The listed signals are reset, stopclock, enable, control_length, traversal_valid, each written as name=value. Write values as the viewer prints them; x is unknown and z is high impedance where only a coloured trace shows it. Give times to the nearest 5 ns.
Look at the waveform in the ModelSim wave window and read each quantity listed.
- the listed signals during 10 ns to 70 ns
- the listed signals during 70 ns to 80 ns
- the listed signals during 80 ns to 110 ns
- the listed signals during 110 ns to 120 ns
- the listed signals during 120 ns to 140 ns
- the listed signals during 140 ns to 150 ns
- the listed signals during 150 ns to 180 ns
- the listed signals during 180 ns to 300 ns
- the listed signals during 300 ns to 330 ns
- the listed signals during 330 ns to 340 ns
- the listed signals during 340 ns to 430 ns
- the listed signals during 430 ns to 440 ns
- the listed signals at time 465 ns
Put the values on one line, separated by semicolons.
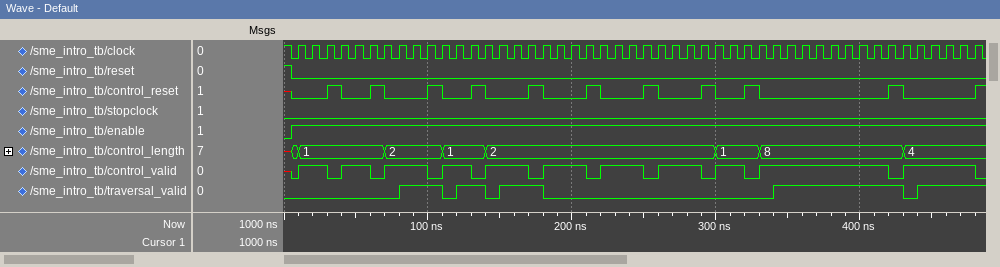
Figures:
reset=0, stopclock=0, enable=1, control_length=1, traversal_valid=0; reset=0, stopclock=0, enable=1, control_length=2, traversal_valid=0; reset=0, stopclock=0, enable=1, control_length=2, traversal_valid=1; reset=0, stopclock=0, enable=1, control_length=1, traversal_valid=0; reset=0, stopclock=0, enable=1, control_length=1, traversal_valid=1; reset=0, stopclock=0, enable=1, control_length=2, traversal_valid=0; reset=0, stopclock=0, enable=1, control_length=2, traversal_valid=1; reset=0, stopclock=0, enable=1, control_length=2, traversal_valid=0; reset=0, stopclock=0, enable=1, control_length=1, traversal_valid=0; reset=0, stopclock=0, enable=1, control_length=8, traversal_valid=0; reset=0, stopclock=0, enable=1, control_length=8, traversal_valid=1; reset=0, stopclock=0, enable=1, control_length=4, traversal_valid=0; reset=0, stopclock=0, enable=1, control_length=4, traversal_valid=1
